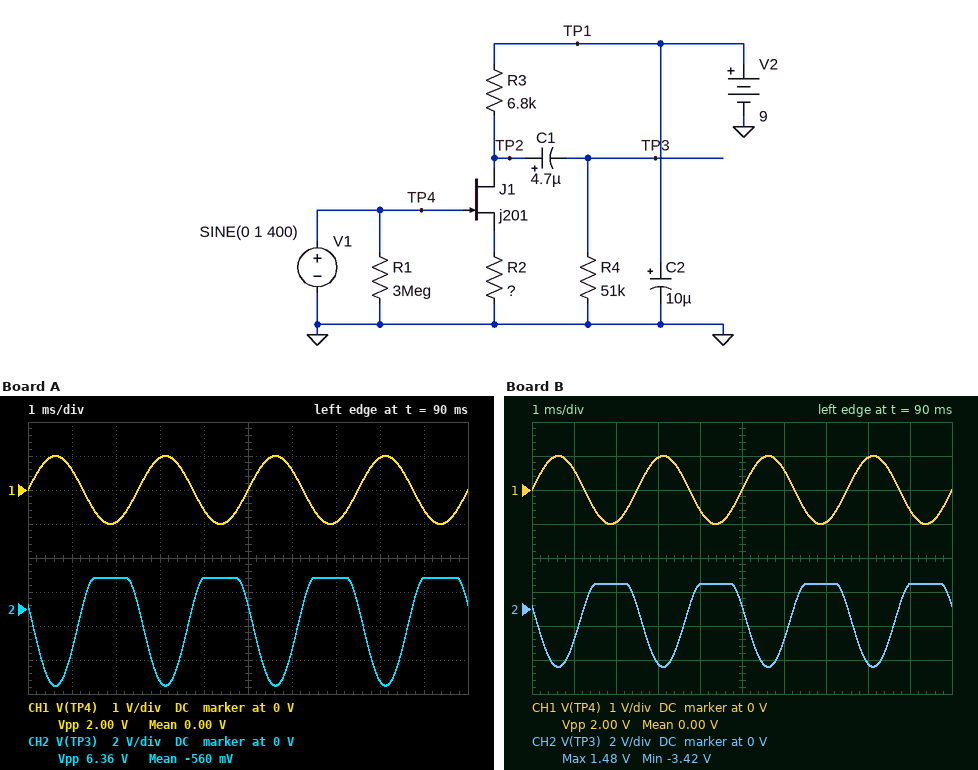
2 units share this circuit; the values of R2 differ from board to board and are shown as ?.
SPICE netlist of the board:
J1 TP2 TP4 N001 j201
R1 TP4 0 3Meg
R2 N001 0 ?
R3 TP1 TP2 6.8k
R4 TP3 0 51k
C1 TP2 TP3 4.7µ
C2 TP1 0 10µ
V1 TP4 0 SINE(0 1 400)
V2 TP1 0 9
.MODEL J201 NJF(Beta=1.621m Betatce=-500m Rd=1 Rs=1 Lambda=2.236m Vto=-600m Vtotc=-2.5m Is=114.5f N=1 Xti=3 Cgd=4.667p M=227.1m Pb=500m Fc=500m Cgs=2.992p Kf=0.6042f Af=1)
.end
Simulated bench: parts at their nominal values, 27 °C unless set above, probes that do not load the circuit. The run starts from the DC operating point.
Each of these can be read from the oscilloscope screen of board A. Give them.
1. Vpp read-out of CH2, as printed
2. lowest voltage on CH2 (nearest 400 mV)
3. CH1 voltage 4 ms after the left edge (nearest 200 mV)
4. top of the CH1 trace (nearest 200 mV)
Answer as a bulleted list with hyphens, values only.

- 6.36 V
- -4.4 V
- -600 mV
- 1.0 V
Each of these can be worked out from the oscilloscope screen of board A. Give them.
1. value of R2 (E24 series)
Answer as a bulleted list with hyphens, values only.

- 750 Ω
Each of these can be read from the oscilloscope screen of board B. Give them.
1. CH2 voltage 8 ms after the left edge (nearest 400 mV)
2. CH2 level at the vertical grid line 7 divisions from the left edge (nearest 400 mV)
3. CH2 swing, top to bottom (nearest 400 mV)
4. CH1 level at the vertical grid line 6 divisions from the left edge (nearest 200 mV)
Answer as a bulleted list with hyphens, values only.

- -3.2 V
- 1.6 V
- 4.8 V
- 600 mV
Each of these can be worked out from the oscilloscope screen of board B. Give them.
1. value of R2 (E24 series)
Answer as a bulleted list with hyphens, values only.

- 1.1 kΩ
